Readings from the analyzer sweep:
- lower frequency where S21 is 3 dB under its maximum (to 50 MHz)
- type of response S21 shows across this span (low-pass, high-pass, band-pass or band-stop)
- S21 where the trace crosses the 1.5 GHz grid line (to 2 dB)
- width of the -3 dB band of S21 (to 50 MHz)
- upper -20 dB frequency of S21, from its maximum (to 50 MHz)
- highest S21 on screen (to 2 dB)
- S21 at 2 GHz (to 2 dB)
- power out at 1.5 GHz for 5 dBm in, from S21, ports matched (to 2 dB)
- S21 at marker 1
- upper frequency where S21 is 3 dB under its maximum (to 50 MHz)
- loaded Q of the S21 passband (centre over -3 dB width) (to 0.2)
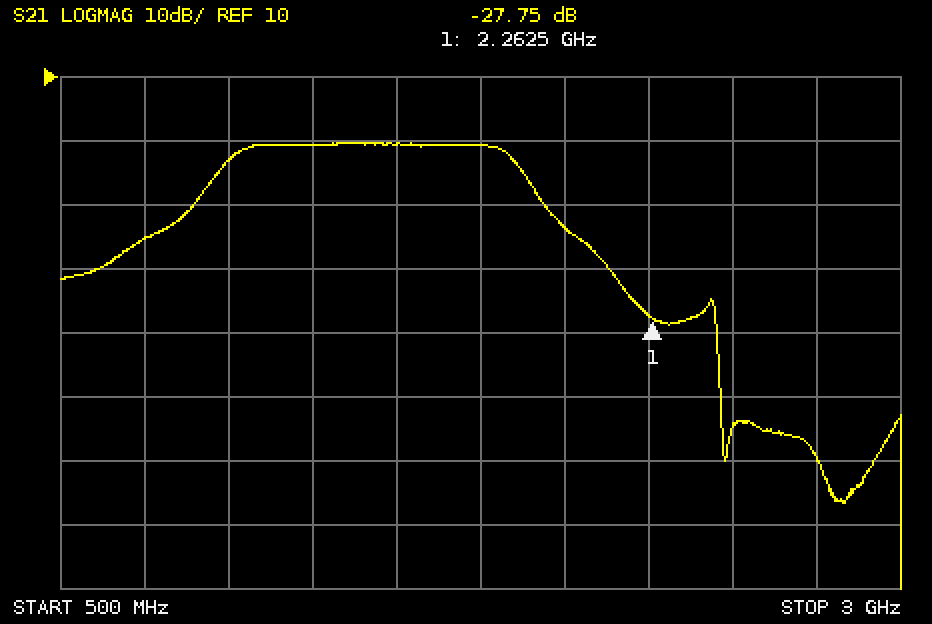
1.00 GHz
band-pass
0 dB
850 MHz
2.15 GHz
0 dB
-14 dB
4 dBm
-27.75 dB
1.85 GHz
1.6
